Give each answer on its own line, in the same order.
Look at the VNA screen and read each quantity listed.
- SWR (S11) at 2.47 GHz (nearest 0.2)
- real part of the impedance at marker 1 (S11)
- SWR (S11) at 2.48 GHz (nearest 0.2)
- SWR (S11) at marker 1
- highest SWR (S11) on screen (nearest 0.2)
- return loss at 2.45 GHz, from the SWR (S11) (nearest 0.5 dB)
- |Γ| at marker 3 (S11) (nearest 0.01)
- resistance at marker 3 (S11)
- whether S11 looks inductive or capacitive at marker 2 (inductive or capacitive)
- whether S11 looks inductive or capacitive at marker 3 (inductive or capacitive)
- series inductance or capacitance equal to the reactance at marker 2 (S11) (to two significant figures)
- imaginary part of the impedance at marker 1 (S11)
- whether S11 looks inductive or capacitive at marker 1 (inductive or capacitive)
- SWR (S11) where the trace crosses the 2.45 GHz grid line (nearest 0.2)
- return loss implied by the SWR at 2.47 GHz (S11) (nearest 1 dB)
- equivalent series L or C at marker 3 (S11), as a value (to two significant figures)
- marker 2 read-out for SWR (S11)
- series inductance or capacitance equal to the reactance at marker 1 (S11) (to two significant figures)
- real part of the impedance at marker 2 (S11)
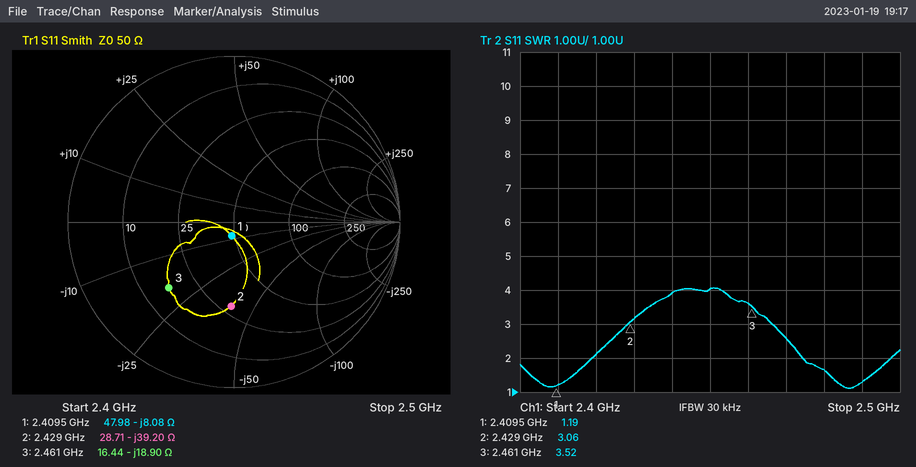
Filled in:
2.6
47.98 Ω
1.6
1.19
4.0
4.5 dB
0.56
16.44 Ω
capacitive
capacitive
1.7 pF
-8.08 Ω
capacitive
4.0
7 dB
3.4 pF
3.06
8.2 pF
28.71 Ω
